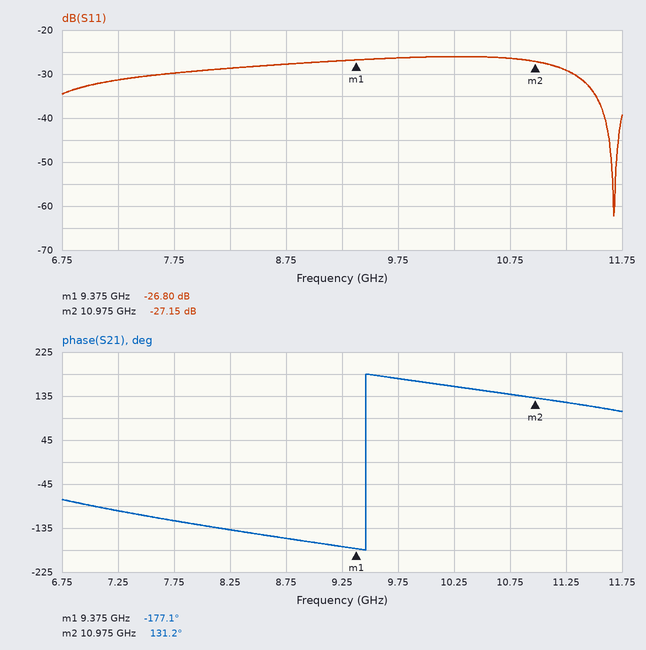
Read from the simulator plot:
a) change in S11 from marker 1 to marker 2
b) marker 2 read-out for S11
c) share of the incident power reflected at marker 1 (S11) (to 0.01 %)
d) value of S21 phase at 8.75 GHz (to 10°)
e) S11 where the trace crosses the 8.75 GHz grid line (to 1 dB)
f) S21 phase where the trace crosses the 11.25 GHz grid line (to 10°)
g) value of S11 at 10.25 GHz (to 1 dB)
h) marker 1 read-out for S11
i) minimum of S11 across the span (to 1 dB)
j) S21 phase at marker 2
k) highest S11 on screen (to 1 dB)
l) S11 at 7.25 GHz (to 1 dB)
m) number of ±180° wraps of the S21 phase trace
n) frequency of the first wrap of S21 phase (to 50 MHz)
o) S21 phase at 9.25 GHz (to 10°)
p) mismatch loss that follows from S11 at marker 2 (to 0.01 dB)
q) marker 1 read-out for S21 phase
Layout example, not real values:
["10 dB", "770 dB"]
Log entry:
["-0.35 dB", "-27.15 dB", "0.21 %", "-160°", "-28 dB", "120°", "-26 dB", "-26.80 dB", "-62 dB", "131.2°", "-26 dB", "-31 dB", "1", "9.45 GHz", "-170°", "0.01 dB", "-177.1°"]
